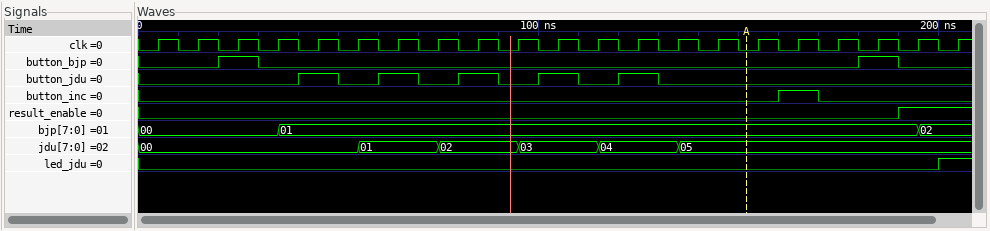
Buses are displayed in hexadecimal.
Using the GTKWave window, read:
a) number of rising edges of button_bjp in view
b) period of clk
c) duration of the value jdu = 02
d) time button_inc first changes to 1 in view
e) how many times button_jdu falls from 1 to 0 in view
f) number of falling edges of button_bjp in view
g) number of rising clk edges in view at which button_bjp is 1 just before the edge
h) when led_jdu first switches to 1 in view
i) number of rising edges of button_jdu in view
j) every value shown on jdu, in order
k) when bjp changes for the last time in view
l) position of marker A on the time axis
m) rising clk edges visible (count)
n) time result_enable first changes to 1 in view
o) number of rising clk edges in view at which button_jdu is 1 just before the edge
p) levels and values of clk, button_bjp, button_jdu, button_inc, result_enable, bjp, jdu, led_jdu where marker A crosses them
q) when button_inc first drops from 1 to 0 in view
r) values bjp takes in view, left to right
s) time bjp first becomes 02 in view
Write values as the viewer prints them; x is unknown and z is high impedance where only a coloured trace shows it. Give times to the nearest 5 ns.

2
10 ns
20 ns
160 ns
5
2
2
200 ns
5
00, 01, 02, 03, 04, 05
195 ns
150 ns
21
190 ns
5
clk=0, button_bjp=0, button_jdu=0, button_inc=0, result_enable=0, bjp=01, jdu=05, led_jdu=0
170 ns
00, 01, 02
195 ns
